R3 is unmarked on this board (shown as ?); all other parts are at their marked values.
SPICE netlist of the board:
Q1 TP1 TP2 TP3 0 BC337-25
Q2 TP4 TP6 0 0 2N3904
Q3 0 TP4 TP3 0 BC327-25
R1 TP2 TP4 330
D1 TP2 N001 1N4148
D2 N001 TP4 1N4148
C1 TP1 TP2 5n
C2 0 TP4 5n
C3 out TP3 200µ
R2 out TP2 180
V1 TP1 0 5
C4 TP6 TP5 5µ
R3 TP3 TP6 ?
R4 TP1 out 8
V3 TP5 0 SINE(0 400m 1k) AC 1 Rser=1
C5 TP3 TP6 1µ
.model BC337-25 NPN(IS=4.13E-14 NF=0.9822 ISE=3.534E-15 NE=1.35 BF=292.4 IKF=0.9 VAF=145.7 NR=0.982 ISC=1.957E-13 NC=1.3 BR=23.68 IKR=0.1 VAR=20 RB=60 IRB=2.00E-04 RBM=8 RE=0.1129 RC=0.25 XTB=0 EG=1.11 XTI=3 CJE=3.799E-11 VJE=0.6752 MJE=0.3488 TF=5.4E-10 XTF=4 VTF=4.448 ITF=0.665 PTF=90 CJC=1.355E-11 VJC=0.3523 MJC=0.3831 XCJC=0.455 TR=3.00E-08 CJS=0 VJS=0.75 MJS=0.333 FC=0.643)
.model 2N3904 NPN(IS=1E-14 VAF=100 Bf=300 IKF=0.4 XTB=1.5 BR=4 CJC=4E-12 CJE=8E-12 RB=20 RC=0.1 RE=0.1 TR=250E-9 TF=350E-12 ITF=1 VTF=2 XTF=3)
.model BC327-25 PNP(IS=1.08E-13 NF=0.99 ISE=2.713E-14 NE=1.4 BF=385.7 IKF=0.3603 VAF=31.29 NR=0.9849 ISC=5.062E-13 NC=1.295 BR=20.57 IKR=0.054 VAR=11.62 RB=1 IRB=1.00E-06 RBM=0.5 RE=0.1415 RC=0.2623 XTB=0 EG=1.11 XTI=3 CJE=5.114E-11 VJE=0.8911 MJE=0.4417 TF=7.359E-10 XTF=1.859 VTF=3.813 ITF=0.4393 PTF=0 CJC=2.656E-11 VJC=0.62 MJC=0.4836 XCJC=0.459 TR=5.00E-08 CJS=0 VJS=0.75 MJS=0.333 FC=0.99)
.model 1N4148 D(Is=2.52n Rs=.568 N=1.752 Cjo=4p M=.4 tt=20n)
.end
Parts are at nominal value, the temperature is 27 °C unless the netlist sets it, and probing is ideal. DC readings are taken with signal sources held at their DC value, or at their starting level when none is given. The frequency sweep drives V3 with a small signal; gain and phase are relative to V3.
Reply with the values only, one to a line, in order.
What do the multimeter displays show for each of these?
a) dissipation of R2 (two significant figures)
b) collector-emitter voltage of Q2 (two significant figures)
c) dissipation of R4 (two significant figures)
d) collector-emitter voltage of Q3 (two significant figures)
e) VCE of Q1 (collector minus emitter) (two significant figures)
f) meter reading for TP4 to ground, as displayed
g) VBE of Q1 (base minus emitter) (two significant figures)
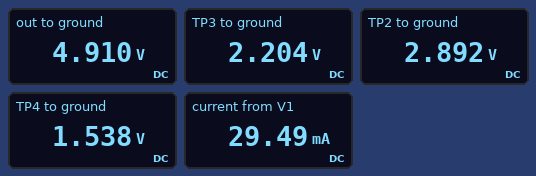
23 mW
1.5 V
1.0 mW
-2.2 V
2.8 V
1.538 V
690 mV
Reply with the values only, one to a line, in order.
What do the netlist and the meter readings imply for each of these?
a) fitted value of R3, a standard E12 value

39 kΩ
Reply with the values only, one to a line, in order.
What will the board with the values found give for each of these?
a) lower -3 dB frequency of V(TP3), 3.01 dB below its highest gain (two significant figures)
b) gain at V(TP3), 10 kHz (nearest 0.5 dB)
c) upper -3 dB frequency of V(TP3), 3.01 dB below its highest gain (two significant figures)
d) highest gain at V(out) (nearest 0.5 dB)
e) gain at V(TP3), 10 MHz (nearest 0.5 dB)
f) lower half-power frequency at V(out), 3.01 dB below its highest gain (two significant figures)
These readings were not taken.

7.2 Hz
13.5 dB
31 kHz
14.0 dB
-6.0 dB
110 Hz
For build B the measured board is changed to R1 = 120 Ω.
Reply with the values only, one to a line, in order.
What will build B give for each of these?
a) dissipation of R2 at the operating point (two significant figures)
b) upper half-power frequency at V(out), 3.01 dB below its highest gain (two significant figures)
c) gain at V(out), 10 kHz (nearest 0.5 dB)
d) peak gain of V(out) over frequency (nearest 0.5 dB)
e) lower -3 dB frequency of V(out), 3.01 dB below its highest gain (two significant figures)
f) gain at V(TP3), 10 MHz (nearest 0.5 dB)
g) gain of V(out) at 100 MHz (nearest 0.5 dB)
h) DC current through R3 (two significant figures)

24 mW
31 kHz
12.5 dB
13.0 dB
95 Hz
-1.5 dB
-2.0 dB
39 µA
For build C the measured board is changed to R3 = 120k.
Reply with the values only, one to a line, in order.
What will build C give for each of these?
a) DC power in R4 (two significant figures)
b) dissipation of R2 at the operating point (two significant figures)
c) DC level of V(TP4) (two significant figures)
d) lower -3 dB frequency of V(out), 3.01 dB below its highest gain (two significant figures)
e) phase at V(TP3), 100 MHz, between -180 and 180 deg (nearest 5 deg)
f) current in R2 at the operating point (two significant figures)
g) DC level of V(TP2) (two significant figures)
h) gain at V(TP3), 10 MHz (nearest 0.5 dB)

310 µW
7.0 mW
2.6 V
100 Hz
-5 deg
6.2 mA
3.8 V
-2.5 dB
